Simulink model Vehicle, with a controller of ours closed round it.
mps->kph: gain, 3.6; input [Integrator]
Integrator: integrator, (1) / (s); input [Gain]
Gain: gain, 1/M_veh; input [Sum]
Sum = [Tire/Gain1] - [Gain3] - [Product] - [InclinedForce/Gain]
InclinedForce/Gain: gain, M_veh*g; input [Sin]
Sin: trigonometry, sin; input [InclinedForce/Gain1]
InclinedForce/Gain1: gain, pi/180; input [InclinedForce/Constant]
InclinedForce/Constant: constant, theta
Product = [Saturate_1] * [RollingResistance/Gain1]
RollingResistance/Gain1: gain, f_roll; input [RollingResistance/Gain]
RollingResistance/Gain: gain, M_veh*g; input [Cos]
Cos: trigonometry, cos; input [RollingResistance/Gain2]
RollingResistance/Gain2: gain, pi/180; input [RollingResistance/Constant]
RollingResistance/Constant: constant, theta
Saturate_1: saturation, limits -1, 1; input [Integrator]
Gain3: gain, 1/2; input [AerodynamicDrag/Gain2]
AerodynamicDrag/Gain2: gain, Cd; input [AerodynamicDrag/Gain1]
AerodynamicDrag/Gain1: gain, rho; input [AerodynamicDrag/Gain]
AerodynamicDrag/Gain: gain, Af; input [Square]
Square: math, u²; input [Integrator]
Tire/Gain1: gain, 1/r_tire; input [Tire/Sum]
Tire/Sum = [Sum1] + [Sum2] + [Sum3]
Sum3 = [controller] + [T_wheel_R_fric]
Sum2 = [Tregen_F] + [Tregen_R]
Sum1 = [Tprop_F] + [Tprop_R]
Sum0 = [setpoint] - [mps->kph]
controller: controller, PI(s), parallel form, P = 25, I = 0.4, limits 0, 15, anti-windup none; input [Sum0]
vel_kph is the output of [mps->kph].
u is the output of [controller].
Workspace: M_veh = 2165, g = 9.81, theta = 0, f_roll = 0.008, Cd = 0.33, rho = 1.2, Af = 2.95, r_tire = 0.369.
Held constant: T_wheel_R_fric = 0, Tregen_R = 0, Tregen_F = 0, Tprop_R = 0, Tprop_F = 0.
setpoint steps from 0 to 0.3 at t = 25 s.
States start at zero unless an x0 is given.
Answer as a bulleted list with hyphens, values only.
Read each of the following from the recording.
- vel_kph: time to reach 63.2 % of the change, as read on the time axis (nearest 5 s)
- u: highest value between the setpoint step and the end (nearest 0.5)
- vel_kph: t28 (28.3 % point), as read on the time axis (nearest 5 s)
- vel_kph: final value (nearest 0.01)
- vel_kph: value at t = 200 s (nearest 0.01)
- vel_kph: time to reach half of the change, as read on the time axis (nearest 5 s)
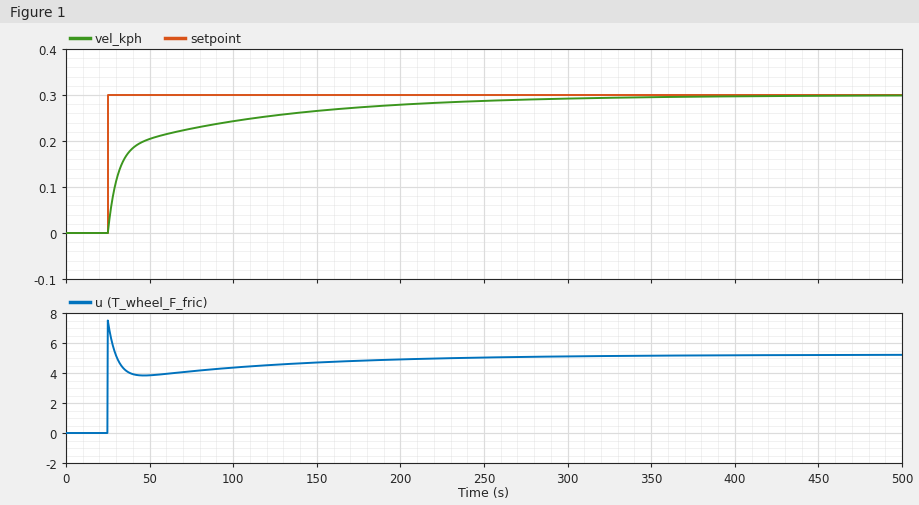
- 40 s
- 7.5
- 30 s
- 0.30
- 0.28
- 35 s
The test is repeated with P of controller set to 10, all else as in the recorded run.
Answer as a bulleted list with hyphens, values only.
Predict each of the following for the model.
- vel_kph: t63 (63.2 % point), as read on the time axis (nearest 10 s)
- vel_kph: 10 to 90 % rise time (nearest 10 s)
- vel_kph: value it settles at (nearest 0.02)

- 60 s
- 110 s
- 0.30
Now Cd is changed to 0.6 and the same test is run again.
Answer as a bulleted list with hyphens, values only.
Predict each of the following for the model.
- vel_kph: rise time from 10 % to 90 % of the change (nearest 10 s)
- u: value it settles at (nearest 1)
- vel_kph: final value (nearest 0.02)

- 140 s
- 5
- 0.30
